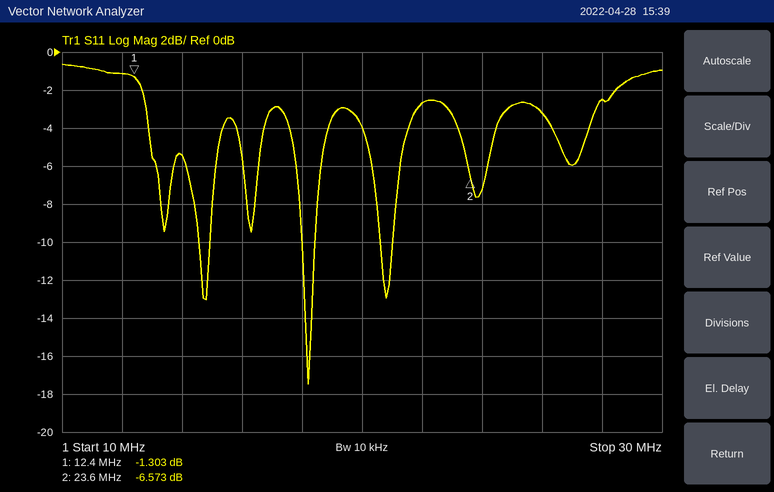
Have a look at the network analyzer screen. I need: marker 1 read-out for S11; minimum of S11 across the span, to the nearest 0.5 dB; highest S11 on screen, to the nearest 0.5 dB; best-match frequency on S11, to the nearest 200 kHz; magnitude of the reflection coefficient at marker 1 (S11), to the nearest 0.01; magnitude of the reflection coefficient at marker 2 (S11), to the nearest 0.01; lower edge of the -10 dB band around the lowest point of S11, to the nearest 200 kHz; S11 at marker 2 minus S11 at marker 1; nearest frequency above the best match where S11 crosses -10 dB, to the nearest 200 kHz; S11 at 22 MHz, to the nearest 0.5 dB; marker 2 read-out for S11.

-1.303 dB
-17.5 dB
-0.5 dB
18.2 MHz
0.86
0.47
18.0 MHz
-5.270 dB
18.4 MHz
-2.5 dB
-6.573 dB
